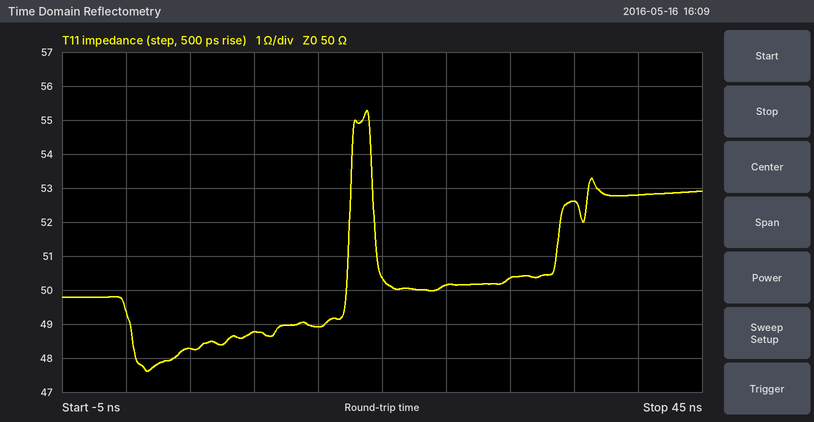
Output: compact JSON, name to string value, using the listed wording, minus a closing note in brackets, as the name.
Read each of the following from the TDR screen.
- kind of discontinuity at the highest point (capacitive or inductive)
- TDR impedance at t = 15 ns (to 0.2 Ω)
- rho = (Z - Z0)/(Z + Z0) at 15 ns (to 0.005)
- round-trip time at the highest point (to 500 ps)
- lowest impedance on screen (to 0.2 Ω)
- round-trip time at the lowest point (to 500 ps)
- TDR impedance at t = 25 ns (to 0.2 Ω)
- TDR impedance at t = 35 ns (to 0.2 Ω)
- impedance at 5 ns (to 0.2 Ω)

{"kind of discontinuity at the highest point": "inductive", "TDR impedance at t = 15 ns": "49.0 Ω", "rho = (Z - Z0)/(Z + Z0) at 15 ns": "-0.010", "round-trip time at the highest point": "19.0 ns", "lowest impedance on screen": "47.6 Ω", "round-trip time at the lowest point": "1.5 ns", "TDR impedance at t = 25 ns": "50.2 Ω", "TDR impedance at t = 35 ns": "52.6 Ω", "impedance at 5 ns": "48.2 Ω"}
